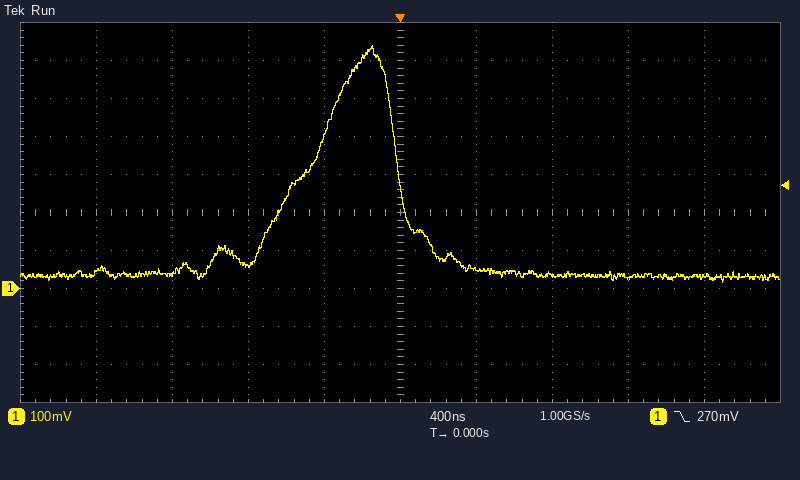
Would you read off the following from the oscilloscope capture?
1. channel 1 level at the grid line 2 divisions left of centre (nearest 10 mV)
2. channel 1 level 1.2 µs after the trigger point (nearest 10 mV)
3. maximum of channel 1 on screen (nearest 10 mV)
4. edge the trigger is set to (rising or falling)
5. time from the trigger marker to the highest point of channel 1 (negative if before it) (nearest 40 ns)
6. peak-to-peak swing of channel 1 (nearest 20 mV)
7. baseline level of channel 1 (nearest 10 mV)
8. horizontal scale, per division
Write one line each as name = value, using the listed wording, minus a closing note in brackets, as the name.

channel 1 level at the grid line 2 divisions left of centre = 60 mV
channel 1 level 1.2 µs after the trigger point = 30 mV
maximum of channel 1 on screen = 640 mV
edge the trigger is set to = falling
time from the trigger marker to the highest point of channel 1 (negative if before it) = -160 ns
peak-to-peak swing of channel 1 = 620 mV
baseline level of channel 1 = 30 mV
horizontal scale, per division = 400 ns
